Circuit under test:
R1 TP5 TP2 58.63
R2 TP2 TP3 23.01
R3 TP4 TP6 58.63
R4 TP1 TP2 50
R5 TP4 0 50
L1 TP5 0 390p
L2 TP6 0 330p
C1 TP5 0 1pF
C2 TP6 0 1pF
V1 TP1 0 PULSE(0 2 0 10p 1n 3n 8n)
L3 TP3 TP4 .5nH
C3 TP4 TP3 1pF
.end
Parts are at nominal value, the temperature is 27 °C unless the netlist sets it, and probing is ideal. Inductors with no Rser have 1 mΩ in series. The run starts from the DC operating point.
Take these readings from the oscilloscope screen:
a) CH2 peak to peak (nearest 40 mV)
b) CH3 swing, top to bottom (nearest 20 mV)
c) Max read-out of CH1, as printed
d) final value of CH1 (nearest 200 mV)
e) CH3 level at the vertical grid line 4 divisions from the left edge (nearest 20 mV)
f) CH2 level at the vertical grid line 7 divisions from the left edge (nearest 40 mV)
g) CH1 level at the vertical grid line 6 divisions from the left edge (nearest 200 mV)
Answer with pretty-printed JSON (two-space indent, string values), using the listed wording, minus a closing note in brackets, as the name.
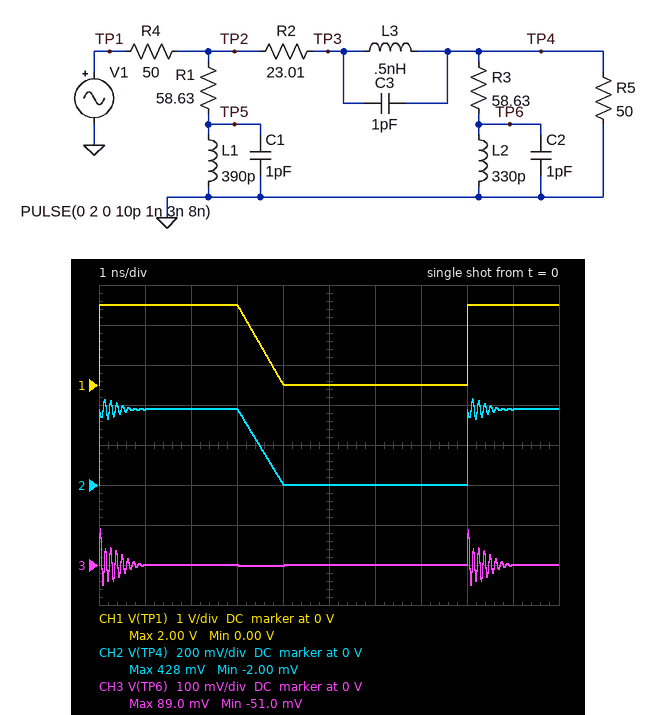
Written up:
{
  "CH2 peak to peak": "440 mV",
  "CH3 swing, top to bottom": "140 mV",
  "Max read-out of CH1, as printed": "2.00 V",
  "final value of CH1": "2.0 V",
  "CH3 level at the vertical grid line 4 divisions from the left edge": "0 V",
  "CH2 level at the vertical grid line 7 divisions from the left edge": "0 V",
  "CH1 level at the vertical grid line 6 divisions from the left edge": "0 V"
}
